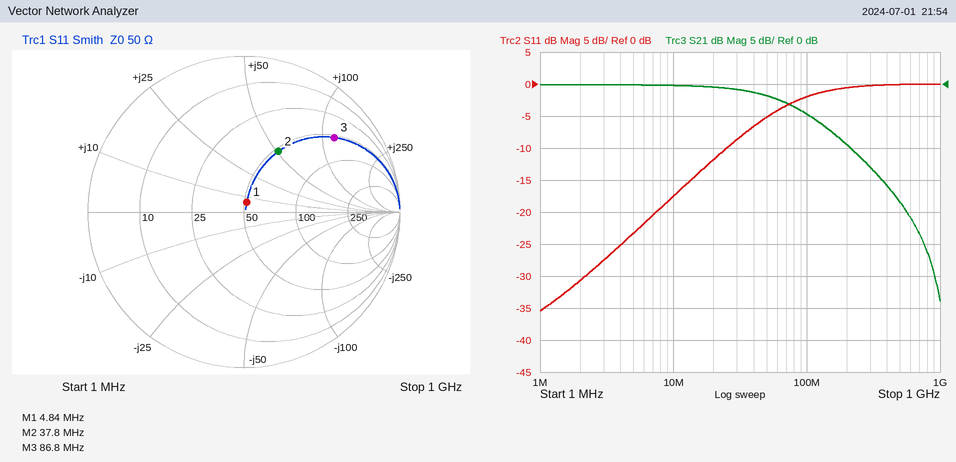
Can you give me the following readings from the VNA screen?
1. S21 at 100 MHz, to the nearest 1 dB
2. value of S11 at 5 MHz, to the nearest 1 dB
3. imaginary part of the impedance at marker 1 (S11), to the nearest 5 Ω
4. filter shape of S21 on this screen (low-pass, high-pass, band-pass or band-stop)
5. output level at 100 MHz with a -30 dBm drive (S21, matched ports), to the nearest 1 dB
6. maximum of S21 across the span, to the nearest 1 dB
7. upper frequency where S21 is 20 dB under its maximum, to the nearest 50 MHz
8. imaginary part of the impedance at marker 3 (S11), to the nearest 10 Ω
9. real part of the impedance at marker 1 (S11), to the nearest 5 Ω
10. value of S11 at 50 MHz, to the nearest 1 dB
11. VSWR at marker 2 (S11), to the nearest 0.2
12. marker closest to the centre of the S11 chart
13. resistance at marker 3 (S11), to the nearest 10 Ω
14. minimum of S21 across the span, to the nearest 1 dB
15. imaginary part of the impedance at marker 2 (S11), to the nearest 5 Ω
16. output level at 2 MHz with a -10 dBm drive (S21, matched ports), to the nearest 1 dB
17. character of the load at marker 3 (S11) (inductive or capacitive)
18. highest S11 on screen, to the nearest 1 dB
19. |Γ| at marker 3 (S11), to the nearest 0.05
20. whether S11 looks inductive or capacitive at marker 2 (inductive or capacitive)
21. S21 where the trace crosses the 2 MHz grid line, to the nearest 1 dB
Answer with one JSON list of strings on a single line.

["-5 dB", "-23 dB", "+5 Ω", "low-pass", "-35 dBm", "0 dB", "550 MHz", "+120 Ω", "50 Ω", "-5 dB", "2.6", "marker 1", "50 Ω", "-34 dB", "+50 Ω", "-10 dBm", "inductive", "0 dB", "0.75", "inductive", "0 dB"]
